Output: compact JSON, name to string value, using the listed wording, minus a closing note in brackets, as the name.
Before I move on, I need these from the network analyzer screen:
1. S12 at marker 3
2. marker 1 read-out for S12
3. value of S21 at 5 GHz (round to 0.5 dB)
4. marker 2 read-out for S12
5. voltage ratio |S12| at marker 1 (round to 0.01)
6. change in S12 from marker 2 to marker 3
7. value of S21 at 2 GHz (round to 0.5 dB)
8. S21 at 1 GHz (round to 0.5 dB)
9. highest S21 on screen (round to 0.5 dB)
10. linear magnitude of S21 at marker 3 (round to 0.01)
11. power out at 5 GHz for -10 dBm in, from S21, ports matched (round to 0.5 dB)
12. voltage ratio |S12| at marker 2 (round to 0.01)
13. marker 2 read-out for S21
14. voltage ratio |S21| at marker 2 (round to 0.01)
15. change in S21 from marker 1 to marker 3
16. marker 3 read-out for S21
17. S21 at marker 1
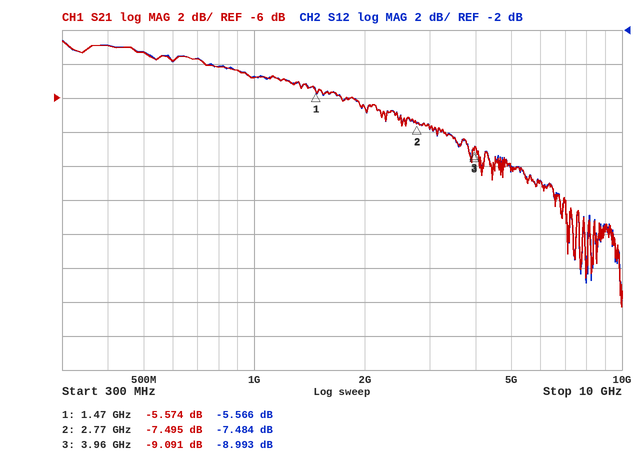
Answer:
{"S12 at marker 3": "-8.993 dB", "marker 1 read-out for S12": "-5.566 dB", "value of S21 at 5 GHz": "-10.0 dB", "marker 2 read-out for S12": "-7.484 dB", "voltage ratio |S12| at marker 1": "0.53", "change in S12 from marker 2 to marker 3": "-1.509 dB", "value of S21 at 2 GHz": "-6.5 dB", "S21 at 1 GHz": "-5.0 dB", "highest S21 on screen": "-2.5 dB", "linear magnitude of S21 at marker 3": "0.35", "power out at 5 GHz for -10 dBm in, from S21, ports matched": "-20.0 dBm", "voltage ratio |S12| at marker 2": "0.42", "marker 2 read-out for S21": "-7.495 dB", "voltage ratio |S21| at marker 2": "0.42", "change in S21 from marker 1 to marker 3": "-3.517 dB", "marker 3 read-out for S21": "-9.091 dB", "S21 at marker 1": "-5.574 dB"}
